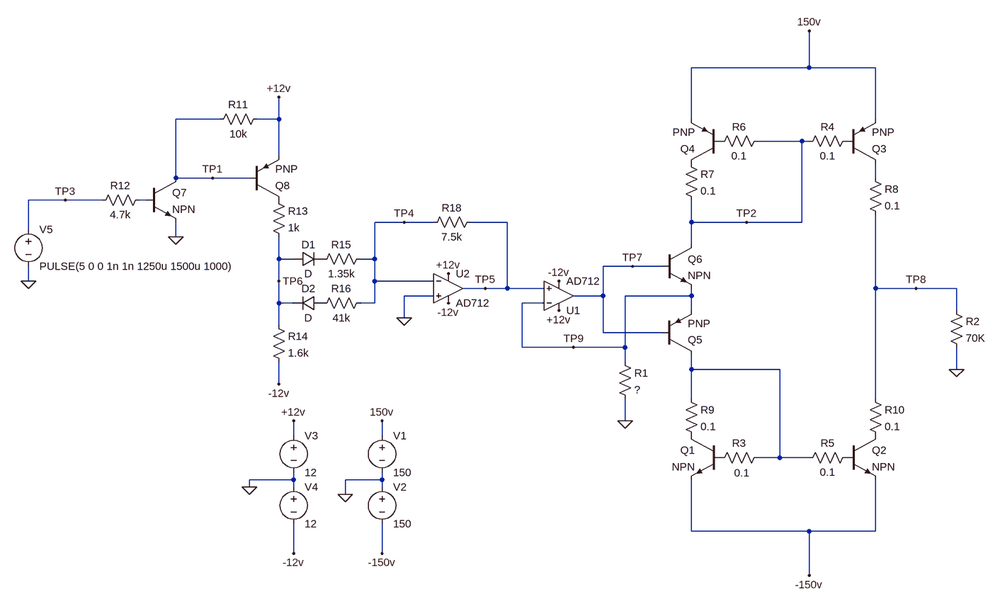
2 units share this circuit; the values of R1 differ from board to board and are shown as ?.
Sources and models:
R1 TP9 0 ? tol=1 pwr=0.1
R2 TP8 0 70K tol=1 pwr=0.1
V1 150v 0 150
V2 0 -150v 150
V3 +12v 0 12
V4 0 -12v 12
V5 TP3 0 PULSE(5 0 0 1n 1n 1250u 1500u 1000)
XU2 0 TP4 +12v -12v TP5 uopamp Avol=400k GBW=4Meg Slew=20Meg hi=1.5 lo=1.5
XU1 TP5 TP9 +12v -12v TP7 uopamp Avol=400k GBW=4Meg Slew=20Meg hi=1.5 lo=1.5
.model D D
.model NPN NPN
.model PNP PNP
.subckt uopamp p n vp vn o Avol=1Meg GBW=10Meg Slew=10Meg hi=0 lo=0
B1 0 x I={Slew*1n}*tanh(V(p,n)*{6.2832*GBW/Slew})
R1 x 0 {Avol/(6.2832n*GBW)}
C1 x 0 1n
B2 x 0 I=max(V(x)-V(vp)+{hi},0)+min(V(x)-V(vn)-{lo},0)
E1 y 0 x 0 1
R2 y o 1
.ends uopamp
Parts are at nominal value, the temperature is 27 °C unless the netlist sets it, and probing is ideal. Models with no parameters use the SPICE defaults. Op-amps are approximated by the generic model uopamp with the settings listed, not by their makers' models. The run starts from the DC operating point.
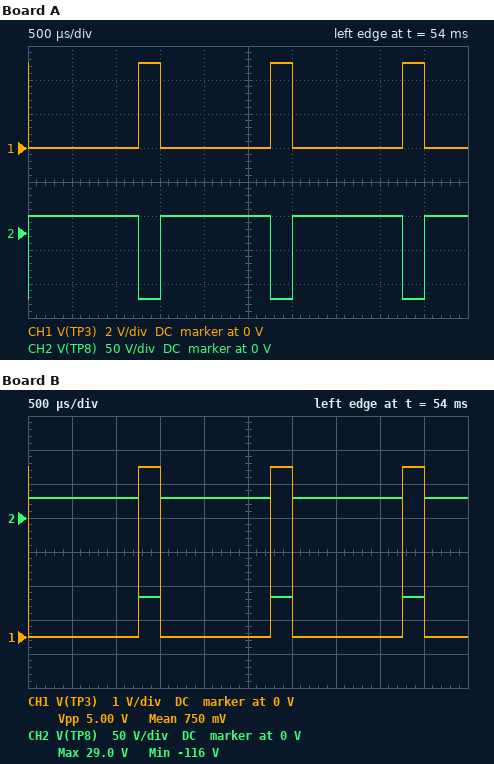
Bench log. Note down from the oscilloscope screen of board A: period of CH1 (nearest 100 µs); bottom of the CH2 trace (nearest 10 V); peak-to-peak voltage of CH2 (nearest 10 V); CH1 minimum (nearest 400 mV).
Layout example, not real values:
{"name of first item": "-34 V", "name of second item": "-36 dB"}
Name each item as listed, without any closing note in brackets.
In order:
{"period of CH1": "1.5 ms", "bottom of the CH2 trace": "-100 V", "peak-to-peak voltage of CH2": "120 V", "CH1 minimum": "0 V"}
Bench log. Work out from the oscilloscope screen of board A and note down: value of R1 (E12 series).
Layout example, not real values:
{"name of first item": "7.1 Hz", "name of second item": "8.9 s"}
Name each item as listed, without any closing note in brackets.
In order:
{"value of R1": "5.6 kΩ"}
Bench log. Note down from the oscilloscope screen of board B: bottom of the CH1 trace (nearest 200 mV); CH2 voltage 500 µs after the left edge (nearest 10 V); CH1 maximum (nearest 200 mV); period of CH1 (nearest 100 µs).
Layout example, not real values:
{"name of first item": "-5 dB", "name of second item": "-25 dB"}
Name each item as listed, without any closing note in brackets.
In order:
{"bottom of the CH1 trace": "0 V", "CH2 voltage 500 µs after the left edge": "30 V", "CH1 maximum": "5.0 V", "period of CH1": "1.5 ms"}
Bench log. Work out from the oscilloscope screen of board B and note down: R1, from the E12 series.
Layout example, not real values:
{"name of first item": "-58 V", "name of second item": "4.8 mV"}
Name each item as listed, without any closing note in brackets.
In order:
{"R1, from the E12 series": "4.7 kΩ"}
